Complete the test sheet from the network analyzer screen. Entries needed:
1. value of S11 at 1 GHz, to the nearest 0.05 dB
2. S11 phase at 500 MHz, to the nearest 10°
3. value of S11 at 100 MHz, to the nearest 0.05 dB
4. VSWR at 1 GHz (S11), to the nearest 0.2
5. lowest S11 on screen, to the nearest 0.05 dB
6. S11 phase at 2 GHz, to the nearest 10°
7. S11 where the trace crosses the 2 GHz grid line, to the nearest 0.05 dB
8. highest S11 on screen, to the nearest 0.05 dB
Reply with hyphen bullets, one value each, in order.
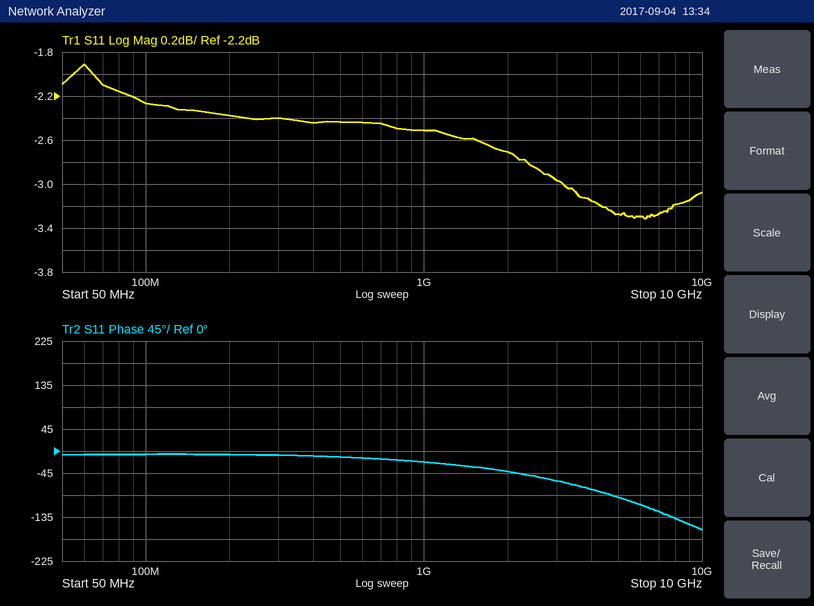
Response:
- -2.50 dB
- -10°
- -2.25 dB
- 7.0
- -3.30 dB
- -40°
- -2.70 dB
- -1.90 dB
